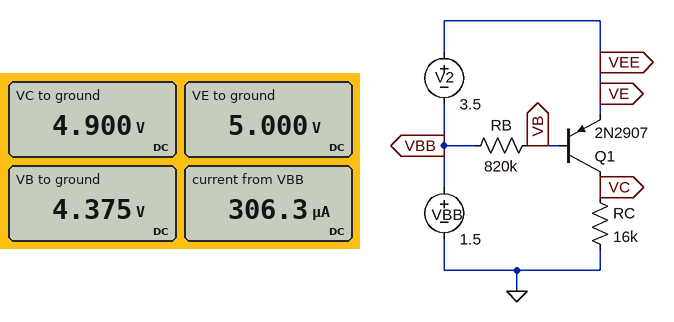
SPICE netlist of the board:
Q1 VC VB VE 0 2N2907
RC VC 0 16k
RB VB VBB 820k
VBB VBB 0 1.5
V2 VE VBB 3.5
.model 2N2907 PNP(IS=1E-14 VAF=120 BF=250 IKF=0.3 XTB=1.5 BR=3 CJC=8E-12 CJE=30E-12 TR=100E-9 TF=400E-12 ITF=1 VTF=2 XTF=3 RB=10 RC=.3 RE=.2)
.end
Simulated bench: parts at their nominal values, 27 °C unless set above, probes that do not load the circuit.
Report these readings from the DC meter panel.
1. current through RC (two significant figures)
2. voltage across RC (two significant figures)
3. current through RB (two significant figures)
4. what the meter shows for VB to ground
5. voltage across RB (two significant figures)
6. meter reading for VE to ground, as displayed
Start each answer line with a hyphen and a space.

- 310 µA
- 4.9 V
- 3.5 µA
- 4.375 V
- 2.9 V
- 5.000 V
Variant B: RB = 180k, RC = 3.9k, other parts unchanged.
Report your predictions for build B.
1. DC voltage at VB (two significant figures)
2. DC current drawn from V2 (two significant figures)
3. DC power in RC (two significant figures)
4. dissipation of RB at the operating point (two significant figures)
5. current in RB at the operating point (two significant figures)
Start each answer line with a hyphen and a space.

- 4.3 V
- 1.3 mA
- 6.2 mW
- 45 µW
- 16 µA
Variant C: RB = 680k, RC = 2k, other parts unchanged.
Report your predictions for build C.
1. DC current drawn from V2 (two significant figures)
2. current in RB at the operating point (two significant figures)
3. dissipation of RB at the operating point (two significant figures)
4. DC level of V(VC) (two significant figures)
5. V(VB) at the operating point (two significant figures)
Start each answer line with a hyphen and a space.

- 1.1 mA
- 4.2 µA
- 12 µW
- 2.1 V
- 4.3 V
